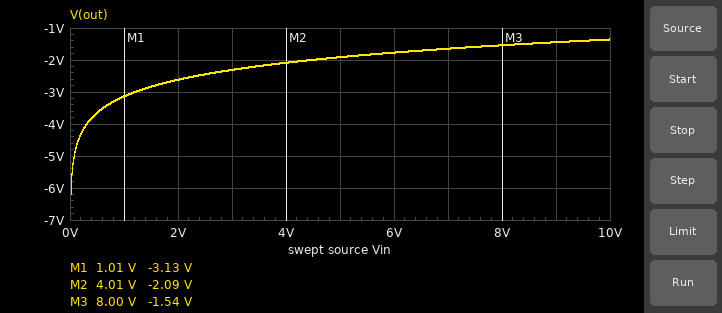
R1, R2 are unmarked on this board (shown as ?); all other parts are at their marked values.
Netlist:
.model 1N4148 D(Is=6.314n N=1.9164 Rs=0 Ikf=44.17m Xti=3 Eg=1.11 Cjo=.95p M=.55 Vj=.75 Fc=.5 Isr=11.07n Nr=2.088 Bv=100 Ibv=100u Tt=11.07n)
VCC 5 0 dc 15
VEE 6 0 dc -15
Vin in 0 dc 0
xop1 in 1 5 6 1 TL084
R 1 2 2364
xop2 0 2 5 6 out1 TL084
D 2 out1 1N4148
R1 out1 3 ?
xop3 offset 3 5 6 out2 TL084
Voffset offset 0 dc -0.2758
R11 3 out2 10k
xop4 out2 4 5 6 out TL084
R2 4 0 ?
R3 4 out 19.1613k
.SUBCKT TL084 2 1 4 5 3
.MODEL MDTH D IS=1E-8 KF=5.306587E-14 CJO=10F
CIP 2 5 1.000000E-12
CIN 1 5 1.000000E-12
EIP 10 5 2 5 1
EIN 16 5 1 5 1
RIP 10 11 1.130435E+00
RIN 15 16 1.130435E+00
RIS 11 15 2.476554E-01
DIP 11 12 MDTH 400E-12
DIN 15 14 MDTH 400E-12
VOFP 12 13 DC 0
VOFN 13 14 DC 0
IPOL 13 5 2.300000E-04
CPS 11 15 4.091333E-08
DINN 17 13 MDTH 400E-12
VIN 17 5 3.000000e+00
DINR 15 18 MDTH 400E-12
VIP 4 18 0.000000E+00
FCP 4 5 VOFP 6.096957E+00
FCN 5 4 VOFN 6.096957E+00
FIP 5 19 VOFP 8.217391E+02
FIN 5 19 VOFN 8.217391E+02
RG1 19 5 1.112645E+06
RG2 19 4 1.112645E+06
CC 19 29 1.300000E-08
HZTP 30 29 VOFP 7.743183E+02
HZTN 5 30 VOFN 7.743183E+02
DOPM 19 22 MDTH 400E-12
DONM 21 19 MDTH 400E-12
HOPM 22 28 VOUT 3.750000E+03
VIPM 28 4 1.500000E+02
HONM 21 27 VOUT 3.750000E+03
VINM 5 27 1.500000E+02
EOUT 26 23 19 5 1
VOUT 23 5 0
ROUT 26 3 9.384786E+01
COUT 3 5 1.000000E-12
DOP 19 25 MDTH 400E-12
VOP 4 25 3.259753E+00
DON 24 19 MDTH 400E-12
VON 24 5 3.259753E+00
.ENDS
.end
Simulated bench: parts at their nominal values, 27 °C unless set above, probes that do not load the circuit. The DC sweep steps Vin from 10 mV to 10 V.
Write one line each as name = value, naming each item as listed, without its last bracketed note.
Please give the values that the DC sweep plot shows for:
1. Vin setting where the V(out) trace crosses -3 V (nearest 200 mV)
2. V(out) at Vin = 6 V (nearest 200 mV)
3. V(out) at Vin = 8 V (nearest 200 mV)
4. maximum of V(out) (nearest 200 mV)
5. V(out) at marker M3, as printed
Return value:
Vin setting where the V(out) trace crosses -3 V = 1.2 V
V(out) at Vin = 6 V = -1.8 V
V(out) at Vin = 8 V = -1.6 V
maximum of V(out) = -1.4 V
V(out) at marker M3, as printed = -1.54 V
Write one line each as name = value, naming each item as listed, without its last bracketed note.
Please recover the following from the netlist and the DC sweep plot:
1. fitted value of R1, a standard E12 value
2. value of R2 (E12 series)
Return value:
fitted value of R1, a standard E12 value = 18 kΩ
value of R2 = 820 Ω
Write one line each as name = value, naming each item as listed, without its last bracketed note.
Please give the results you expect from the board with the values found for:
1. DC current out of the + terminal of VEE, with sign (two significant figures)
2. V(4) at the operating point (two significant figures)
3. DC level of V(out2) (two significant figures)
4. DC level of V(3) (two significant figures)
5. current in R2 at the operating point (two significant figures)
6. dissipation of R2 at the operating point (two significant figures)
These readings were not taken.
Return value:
DC current out of the + terminal of VEE, with sign = -6.2 mA
V(4) at the operating point = -430 mV
DC level of V(out2) = -430 mV
DC level of V(3) = -280 mV
current in R2 at the operating point = 520 µA
dissipation of R2 at the operating point = 220 µW
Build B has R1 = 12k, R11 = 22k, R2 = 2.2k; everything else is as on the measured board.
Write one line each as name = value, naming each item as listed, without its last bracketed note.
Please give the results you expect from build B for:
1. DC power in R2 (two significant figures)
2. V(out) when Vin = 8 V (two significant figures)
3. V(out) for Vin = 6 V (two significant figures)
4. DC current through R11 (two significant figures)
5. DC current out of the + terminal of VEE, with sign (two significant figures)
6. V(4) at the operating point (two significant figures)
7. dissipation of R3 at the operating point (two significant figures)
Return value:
DC power in R2 = 280 µW
V(out) when Vin = 8 V = 4.1 V
V(out) for Vin = 6 V = 3.8 V
DC current through R11 = 23 µA
DC current out of the + terminal of VEE, with sign = -6.0 mA
V(4) at the operating point = -780 mV
dissipation of R3 at the operating point = 2.4 mW
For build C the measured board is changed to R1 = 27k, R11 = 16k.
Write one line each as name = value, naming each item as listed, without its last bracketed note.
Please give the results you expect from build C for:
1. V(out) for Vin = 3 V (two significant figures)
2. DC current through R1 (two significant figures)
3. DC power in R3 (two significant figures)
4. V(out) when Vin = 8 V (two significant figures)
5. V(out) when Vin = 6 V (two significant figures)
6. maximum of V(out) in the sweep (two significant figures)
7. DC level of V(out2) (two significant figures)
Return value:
V(out) for Vin = 3 V = -2.0 V
DC current through R1 = 10 µA
DC power in R3 = 5.5 mW
V(out) when Vin = 8 V = -1.2 V
V(out) when Vin = 6 V = -1.4 V
maximum of V(out) in the sweep = -1.0 V
DC level of V(out2) = -440 mV
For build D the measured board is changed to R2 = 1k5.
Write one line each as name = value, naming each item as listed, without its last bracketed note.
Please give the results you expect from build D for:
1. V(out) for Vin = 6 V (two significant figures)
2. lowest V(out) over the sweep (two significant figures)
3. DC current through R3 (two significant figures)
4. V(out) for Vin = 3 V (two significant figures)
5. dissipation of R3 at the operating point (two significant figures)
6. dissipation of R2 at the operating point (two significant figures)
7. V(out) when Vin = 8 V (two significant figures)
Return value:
V(out) for Vin = 6 V = -1.0 V
lowest V(out) over the sweep = -3.7 V
DC current through R3 = 290 µA
V(out) for Vin = 3 V = -1.3 V
dissipation of R3 at the operating point = 1.6 mW
dissipation of R2 at the operating point = 120 µW
V(out) when Vin = 8 V = -870 mV
